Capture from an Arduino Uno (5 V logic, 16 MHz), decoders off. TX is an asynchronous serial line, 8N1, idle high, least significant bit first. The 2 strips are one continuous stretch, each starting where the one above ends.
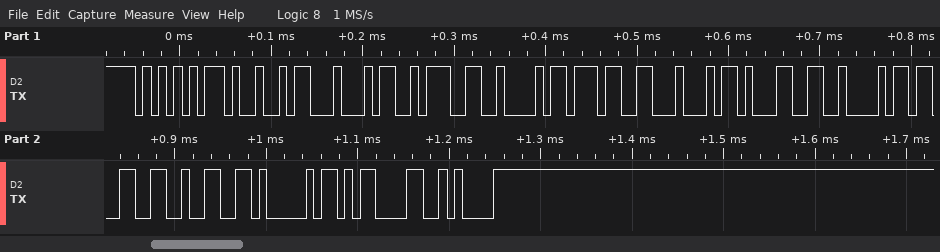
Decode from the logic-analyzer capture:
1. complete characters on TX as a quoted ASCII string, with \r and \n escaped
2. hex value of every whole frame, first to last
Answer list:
"UID:B7D1B32A\r\n"
0x55 0x49 0x44 0x3A 0x42 0x37 0x44 0x31 0x42 0x33 0x32 0x41 0x0D 0x0A
